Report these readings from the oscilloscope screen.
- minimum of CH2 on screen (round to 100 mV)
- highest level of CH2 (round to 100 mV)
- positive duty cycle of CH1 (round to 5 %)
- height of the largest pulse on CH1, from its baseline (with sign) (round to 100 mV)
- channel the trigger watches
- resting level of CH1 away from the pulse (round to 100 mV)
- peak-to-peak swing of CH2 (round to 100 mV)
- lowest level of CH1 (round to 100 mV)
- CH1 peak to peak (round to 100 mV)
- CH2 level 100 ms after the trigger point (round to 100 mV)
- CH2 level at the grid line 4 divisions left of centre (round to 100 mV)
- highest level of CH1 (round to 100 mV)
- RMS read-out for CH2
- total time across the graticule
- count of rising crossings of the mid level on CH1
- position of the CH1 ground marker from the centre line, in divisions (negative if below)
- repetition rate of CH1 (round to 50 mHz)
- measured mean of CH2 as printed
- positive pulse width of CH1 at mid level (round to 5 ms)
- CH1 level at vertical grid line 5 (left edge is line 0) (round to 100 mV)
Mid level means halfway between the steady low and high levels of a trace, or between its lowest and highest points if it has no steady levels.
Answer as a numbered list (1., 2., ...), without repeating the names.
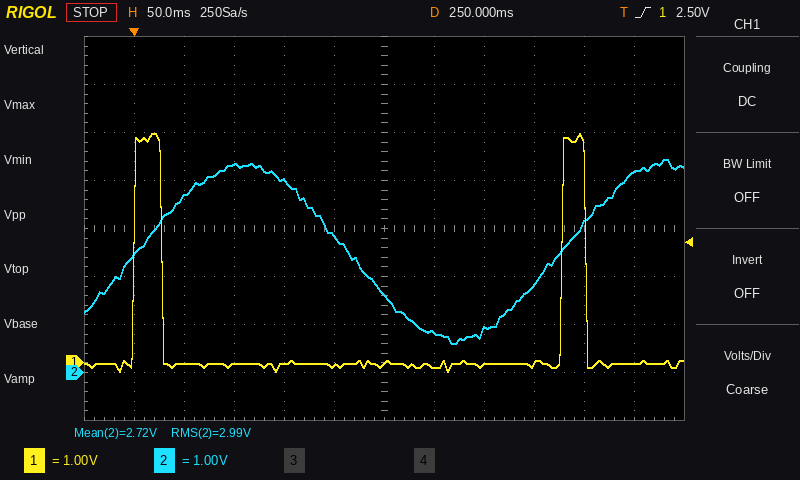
1. 600 mV
2. 4.4 V
3. 5 %
4. +4.8 V
5. CH1
6. 0.0 V
7. 3.8 V
8. -200 mV
9. 5.0 V
10. 4.3 V
11. 3.7 V
12. 4.8 V
13. 2.99 V
14. 600 ms
15. 2
16. -2.8 div
17. 2.35 Hz
18. 2.72 V
19. 25 ms
20. -100 mV
